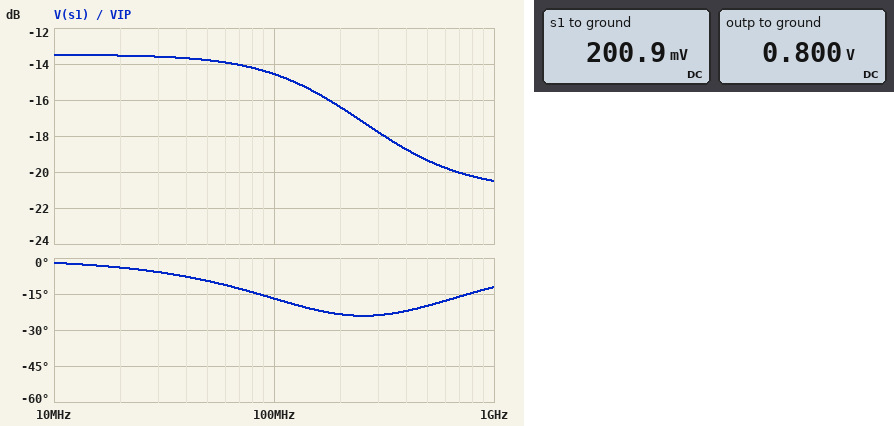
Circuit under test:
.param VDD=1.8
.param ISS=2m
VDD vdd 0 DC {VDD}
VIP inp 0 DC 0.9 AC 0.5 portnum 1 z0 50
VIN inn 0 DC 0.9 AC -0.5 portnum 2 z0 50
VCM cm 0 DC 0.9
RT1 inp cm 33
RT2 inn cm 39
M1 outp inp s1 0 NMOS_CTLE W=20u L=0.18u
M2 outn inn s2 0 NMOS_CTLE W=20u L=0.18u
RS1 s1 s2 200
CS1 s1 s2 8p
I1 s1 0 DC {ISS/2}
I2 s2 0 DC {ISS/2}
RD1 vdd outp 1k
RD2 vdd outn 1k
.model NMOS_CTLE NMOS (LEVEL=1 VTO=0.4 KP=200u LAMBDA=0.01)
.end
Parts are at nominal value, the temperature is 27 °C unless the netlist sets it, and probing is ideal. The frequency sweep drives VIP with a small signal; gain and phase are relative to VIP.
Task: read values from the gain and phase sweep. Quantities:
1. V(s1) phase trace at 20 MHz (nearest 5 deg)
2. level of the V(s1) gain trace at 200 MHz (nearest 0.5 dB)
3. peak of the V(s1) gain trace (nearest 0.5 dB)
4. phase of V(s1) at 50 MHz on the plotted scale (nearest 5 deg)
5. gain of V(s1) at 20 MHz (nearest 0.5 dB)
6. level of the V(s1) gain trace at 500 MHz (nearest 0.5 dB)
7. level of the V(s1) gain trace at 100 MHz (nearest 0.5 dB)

-5 deg
-16.5 dB
-13.5 dB
-10 deg
-13.5 dB
-19.5 dB
-14.5 dB
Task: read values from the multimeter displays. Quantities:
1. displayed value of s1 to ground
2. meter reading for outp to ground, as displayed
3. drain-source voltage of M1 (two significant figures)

200.9 mV
0.800 V
600 mV
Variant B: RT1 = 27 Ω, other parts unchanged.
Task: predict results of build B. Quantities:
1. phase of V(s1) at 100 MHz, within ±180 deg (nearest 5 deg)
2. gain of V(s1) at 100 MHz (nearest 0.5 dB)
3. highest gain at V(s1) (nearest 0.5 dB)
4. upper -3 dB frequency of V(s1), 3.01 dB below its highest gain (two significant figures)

-20 deg
-16.0 dB
-15.0 dB
190 MHz
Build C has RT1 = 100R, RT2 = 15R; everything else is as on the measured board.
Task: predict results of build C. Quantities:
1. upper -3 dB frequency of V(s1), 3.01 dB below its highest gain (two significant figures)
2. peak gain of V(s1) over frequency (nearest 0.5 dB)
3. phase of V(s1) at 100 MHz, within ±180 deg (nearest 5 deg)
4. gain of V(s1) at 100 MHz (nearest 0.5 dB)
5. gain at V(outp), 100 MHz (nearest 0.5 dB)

390 MHz
-7.5 dB
-10 deg
-8.0 dB
5.5 dB
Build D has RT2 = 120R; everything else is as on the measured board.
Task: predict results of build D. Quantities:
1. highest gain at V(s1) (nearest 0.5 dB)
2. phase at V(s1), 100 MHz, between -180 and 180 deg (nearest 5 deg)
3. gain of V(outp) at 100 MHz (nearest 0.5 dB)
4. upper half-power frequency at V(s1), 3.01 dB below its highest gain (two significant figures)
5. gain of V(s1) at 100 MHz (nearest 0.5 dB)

-15.5 dB
-25 deg
5.0 dB
170 MHz
-16.5 dB
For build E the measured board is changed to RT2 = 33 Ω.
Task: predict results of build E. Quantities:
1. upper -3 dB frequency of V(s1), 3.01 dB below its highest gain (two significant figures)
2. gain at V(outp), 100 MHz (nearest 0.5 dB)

220 MHz
3.0 dB
